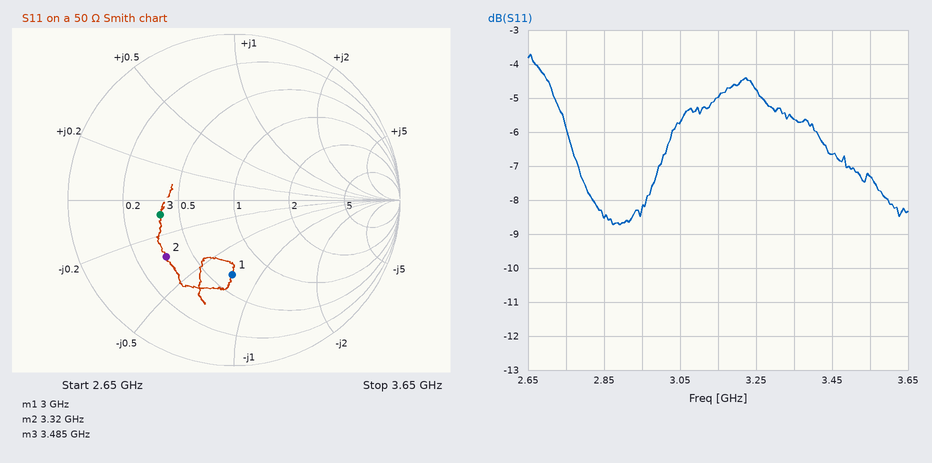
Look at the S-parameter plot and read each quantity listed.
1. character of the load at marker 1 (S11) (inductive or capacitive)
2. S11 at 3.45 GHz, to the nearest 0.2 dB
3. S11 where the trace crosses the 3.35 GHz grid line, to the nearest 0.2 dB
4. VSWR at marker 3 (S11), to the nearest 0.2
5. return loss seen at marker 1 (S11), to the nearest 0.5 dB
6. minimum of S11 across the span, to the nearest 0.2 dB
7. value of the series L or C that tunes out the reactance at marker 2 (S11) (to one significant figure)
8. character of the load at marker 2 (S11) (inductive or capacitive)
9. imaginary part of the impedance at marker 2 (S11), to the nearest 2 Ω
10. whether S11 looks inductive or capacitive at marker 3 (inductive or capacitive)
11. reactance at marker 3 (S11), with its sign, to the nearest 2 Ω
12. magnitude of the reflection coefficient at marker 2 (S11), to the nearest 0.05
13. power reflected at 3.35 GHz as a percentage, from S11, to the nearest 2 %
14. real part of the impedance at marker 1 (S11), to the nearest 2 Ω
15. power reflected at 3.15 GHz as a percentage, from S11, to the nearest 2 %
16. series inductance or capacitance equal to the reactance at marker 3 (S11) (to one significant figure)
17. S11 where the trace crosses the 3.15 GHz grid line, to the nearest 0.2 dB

capacitive
-6.6 dB
-5.6 dB
2.6
7.0 dB
-8.8 dB
800 pH
capacitive
-16 Ω
capacitive
-4 Ω
0.55
28 %
32 Ω
32 %
10 pF
-5.0 dB
